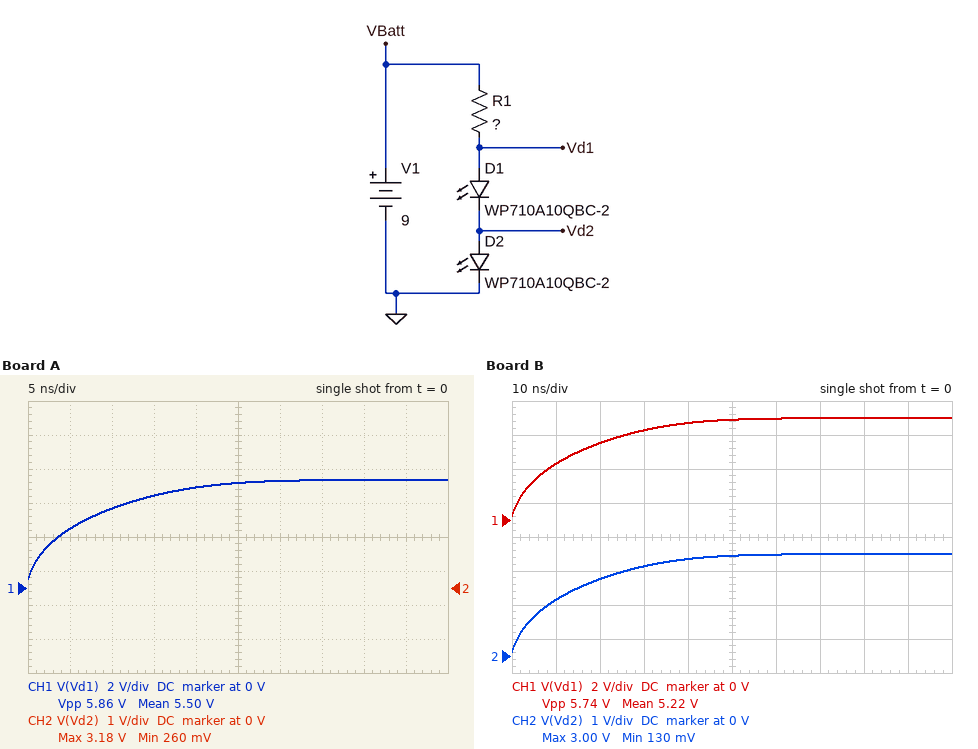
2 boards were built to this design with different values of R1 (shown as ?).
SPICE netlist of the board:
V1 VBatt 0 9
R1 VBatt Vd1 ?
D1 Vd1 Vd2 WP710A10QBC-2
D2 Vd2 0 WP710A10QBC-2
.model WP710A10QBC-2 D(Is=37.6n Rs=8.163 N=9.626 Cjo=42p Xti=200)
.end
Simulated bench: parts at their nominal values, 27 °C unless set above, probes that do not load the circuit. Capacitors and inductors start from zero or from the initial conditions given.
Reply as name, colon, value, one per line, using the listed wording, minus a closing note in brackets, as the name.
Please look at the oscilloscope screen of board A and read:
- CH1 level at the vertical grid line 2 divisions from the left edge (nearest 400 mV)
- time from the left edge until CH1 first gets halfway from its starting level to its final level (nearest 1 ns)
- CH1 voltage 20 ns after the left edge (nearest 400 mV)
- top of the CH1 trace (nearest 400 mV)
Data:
CH1 level at the vertical grid line 2 divisions from the left edge: 4.8 V
time from the left edge until CH1 first gets halfway from its starting level to its final level: 5 ns
CH1 voltage 20 ns after the left edge: 6.0 V
top of the CH1 trace: 6.4 V
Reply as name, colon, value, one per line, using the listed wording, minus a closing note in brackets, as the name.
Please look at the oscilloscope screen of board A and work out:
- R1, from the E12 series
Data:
R1, from the E12 series: 270 Ω
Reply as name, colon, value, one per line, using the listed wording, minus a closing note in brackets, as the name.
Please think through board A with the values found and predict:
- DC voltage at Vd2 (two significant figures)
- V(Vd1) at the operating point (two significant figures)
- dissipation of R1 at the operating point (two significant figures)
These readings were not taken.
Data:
DC voltage at Vd2: 3.2 V
V(Vd1) at the operating point: 6.4 V
dissipation of R1 at the operating point: 26 mW
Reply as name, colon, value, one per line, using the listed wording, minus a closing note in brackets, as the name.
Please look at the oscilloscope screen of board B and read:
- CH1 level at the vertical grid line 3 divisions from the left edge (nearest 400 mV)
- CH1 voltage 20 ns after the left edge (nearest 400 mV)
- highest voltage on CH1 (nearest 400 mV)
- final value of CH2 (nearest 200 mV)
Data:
CH1 level at the vertical grid line 3 divisions from the left edge: 5.2 V
CH1 voltage 20 ns after the left edge: 4.4 V
highest voltage on CH1: 6.0 V
final value of CH2: 3.0 V
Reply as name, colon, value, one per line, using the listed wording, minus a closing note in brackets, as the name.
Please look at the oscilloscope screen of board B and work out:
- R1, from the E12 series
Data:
R1, from the E12 series: 560 Ω
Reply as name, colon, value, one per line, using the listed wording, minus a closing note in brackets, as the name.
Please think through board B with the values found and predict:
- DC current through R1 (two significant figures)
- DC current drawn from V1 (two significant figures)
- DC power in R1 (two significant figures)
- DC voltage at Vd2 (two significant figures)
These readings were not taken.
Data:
DC current through R1: 5.4 mA
DC current drawn from V1: 5.4 mA
DC power in R1: 16 mW
DC voltage at Vd2: 3.0 V
